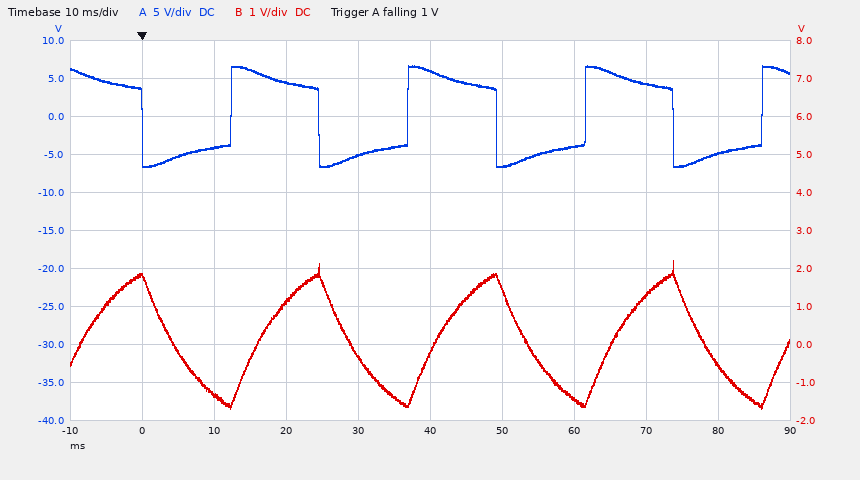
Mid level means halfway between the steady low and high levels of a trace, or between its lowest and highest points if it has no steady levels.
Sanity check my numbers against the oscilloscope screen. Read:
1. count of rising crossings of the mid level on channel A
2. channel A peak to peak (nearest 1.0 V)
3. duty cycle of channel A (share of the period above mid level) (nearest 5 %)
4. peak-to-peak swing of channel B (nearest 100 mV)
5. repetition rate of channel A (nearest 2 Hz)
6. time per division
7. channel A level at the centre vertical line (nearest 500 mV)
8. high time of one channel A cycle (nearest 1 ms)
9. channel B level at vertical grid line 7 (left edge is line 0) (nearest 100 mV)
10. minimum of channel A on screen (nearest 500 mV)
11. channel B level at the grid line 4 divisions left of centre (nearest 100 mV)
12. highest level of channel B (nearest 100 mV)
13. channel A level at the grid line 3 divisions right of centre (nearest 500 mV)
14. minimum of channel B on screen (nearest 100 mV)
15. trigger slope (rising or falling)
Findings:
4
13.0 V
50 %
3.9 V
40 Hz
10 ms
6.0 V
12 ms
-1.4 V
-6.5 V
1.8 V
2.2 V
4.5 V
-1.7 V
falling
